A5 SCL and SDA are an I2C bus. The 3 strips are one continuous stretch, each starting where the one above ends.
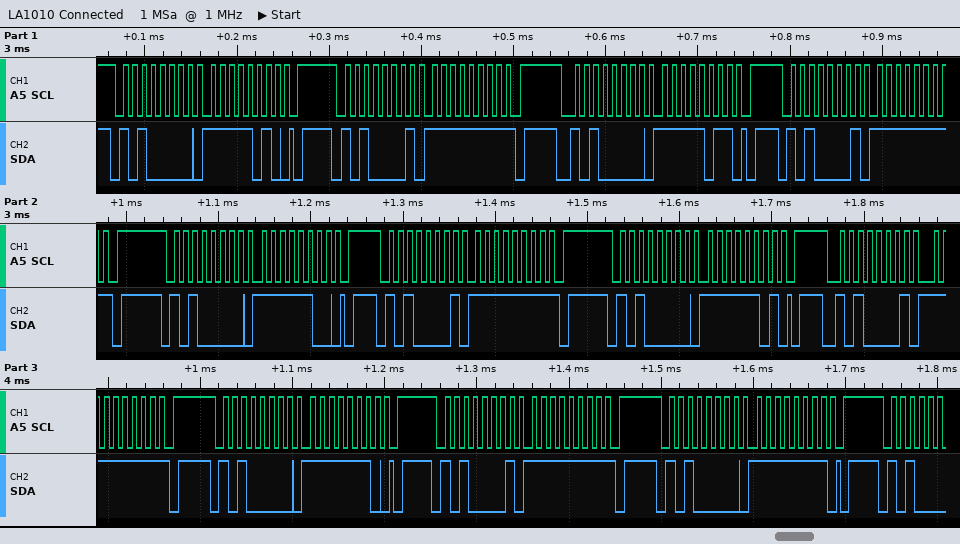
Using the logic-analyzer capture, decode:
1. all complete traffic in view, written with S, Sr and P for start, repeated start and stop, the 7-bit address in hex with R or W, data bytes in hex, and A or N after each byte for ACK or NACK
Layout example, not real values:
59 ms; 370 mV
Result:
S 50W A FA A P S 50R A FF N P S 50W A FB A P S 50R A FF N P S 50W A FC A P S 50R A FF N P S 50W A FD A P S 50R A FF N P S 50W A FE A P S 50R A FF N P S 50W A FF A P
